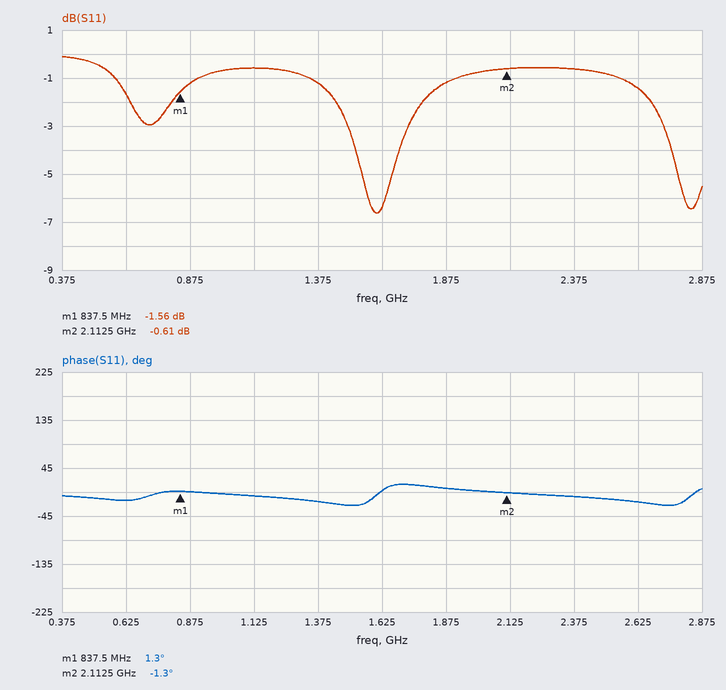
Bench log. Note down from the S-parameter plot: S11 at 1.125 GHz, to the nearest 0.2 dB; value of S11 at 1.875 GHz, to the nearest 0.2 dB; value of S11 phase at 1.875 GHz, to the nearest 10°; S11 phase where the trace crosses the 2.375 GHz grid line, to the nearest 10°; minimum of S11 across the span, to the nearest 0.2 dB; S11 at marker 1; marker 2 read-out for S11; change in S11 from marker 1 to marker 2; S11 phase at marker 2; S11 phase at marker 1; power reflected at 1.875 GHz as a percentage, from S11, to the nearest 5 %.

-0.6 dB
-1.2 dB
10°
-10°
-6.6 dB
-1.56 dB
-0.61 dB
0.95 dB
-1.3°
1.3°
75 %
